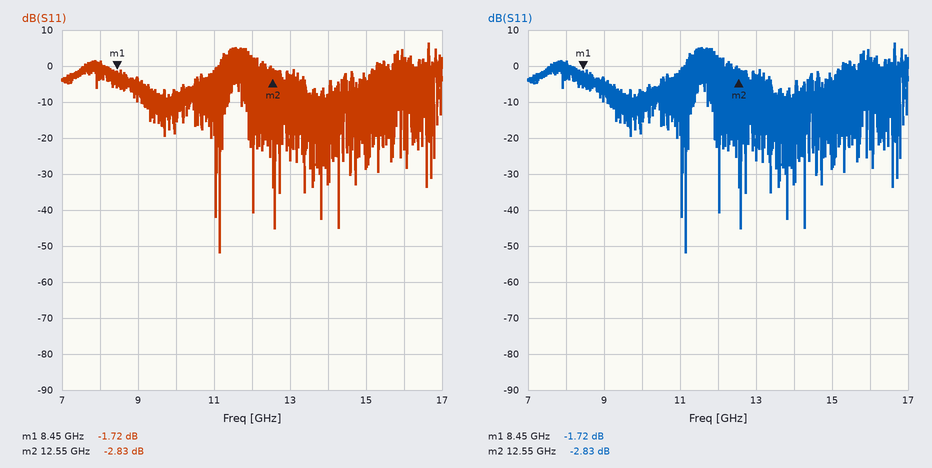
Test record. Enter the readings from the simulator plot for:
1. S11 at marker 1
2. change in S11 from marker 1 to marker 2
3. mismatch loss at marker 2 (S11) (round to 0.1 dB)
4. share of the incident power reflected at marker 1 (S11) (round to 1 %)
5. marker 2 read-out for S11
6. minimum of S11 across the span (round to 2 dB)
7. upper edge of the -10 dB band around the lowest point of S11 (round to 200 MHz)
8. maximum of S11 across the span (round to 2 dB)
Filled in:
-1.72 dB
-1.11 dB
3.2 dB
67 %
-2.83 dB
-52 dB
11.2 GHz
6 dB
